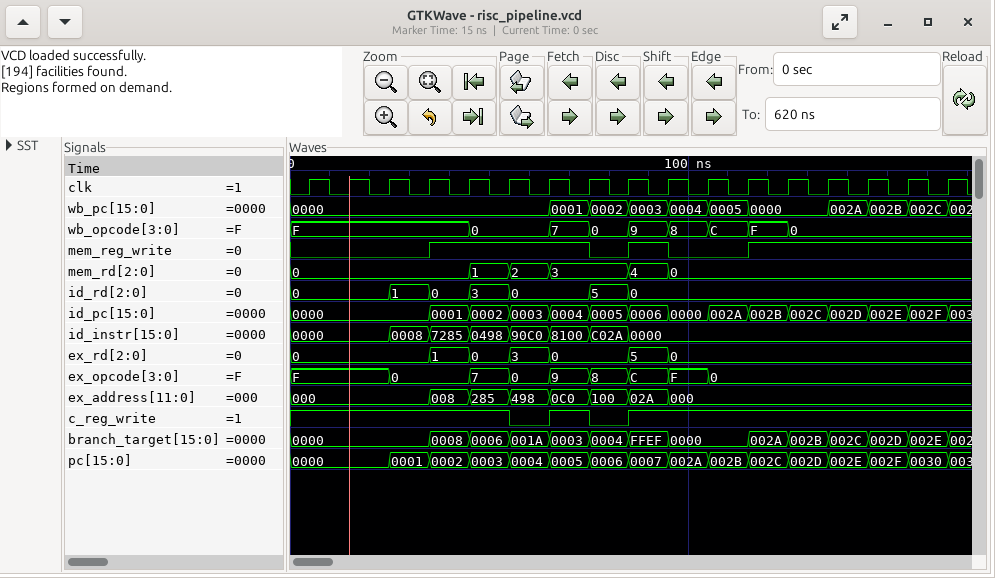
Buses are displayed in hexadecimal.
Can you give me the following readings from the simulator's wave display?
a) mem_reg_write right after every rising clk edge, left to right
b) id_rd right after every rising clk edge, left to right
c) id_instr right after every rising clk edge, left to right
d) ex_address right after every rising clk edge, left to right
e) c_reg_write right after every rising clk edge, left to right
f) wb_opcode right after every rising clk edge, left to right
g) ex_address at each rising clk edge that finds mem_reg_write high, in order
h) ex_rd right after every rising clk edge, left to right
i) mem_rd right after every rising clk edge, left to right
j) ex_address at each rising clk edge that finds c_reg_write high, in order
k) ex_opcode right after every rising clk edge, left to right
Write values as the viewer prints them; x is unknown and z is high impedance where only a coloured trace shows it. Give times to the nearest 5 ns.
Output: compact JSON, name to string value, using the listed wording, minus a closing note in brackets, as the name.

{"mem_reg_write right after every rising clk edge, left to right": "0 0 0 1 1 1 1 0 1 0 0 1 1 1 1 1 1", "id_rd right after every rising clk edge, left to right": "0, 0, 1, 0, 3, 0, 0, 5, 0, 0, 0, 0, 0, 0, 0, 0, 0", "id_instr right after every rising clk edge, left to right": "0000, 0000, 0008, 7285, 0498, 90C0, 8100, C02A, 0000, 0000, 0000, 0000, 0000, 0000, 0000, 0000, 0000", "ex_address right after every rising clk edge, left to right": "000, 000, 000, 008, 285, 498, 0C0, 100, 02A, 000, 000, 000, 000, 000, 000, 000, 000", "c_reg_write right after every rising clk edge, left to right": "1 1 1 1 1 0 1 0 1 1 1 1 1 1 1 1 1", "wb_opcode right after every rising clk edge, left to right": "F, F, F, F, 0, 0, 7, 0, 9, 8, C, F, 0, 0, 0, 0, 0", "ex_address at each rising clk edge that finds mem_reg_write high, in order": "008, 285, 498, 0C0, 02A, 000, 000, 000, 000, 000", "ex_rd right after every rising clk edge, left to right": "0, 0, 0, 1, 0, 3, 0, 0, 5, 0, 0, 0, 0, 0, 0, 0, 0", "mem_rd right after every rising clk edge, left to right": "0, 0, 0, 0, 1, 2, 3, 3, 4, 0, 0, 0, 0, 0, 0, 0, 0", "ex_address at each rising clk edge that finds c_reg_write high, in order": "000, 000, 000, 000, 008, 285, 0C0, 02A, 000, 000, 000, 000, 000, 000, 000", "ex_opcode right after every rising clk edge, left to right": "F, F, 0, 0, 7, 0, 9, 8, C, F, 0, 0, 0, 0, 0, 0, 0"}
